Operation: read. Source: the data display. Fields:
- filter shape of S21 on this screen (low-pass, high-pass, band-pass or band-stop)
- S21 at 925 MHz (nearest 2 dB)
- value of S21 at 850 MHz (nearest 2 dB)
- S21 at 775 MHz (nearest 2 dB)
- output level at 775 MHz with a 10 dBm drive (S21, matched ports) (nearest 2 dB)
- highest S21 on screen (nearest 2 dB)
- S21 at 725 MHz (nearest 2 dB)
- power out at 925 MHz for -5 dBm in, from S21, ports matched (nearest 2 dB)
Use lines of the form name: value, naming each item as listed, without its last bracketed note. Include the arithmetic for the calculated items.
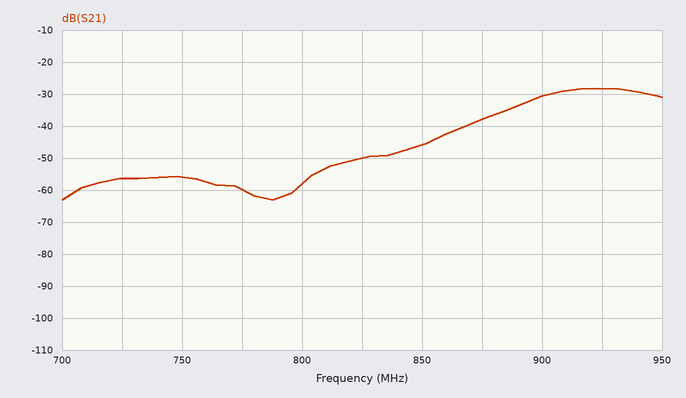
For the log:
filter shape of S21 on this screen: high-pass
S21 at 925 MHz: -28 dB
value of S21 at 850 MHz: -46 dB
S21 at 775 MHz: -60 dB
output level at 775 MHz with a 10 dBm drive (S21, matched ports): 10 dBm + (-60 dB) = -50 dBm
highest S21 on screen: -28 dB
S21 at 725 MHz: -56 dB
power out at 925 MHz for -5 dBm in, from S21, ports matched: -5 dBm + (-28 dB) = -34 dBm
